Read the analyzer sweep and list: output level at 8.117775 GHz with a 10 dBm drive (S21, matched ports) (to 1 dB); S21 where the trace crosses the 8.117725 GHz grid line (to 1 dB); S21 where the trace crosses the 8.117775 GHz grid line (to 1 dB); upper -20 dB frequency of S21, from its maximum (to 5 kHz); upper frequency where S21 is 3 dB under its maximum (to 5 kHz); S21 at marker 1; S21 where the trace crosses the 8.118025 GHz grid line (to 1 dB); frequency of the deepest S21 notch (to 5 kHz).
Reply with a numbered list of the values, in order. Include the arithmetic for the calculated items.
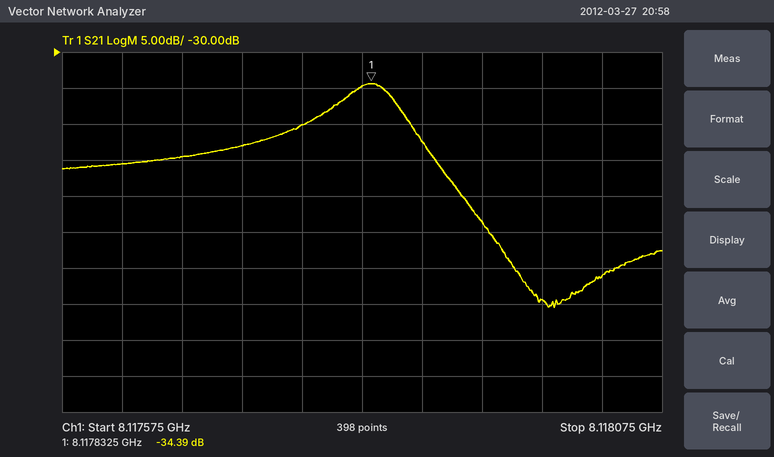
1. 10 dBm + (-40 dB) = -30 dBm
2. -43 dB
3. -40 dB
4. 8.117930 GHz
5. 8.117855 GHz
6. -34.39 dB
7. -61 dB
8. 8.117985 GHz
